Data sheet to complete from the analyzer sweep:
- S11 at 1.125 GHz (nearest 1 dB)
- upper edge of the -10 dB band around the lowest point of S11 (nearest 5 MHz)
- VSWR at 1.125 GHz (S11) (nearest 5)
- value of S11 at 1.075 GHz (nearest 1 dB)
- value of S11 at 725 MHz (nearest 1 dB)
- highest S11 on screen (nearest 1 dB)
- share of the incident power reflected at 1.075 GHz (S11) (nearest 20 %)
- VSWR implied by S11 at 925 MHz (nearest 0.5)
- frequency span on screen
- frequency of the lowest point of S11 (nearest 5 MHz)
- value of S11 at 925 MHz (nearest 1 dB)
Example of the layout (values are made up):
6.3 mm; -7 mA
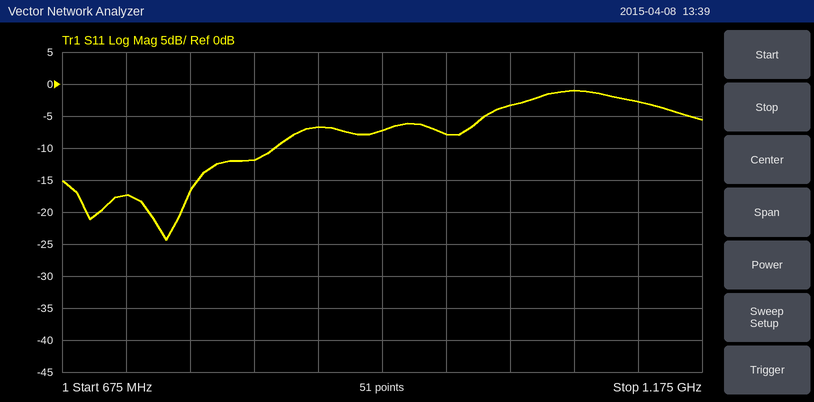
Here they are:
-3 dB; 840 MHz; 5; -1 dB; -17 dB; -1 dB; 80 %; 2.5; 500 MHz; 755 MHz; -7 dB
